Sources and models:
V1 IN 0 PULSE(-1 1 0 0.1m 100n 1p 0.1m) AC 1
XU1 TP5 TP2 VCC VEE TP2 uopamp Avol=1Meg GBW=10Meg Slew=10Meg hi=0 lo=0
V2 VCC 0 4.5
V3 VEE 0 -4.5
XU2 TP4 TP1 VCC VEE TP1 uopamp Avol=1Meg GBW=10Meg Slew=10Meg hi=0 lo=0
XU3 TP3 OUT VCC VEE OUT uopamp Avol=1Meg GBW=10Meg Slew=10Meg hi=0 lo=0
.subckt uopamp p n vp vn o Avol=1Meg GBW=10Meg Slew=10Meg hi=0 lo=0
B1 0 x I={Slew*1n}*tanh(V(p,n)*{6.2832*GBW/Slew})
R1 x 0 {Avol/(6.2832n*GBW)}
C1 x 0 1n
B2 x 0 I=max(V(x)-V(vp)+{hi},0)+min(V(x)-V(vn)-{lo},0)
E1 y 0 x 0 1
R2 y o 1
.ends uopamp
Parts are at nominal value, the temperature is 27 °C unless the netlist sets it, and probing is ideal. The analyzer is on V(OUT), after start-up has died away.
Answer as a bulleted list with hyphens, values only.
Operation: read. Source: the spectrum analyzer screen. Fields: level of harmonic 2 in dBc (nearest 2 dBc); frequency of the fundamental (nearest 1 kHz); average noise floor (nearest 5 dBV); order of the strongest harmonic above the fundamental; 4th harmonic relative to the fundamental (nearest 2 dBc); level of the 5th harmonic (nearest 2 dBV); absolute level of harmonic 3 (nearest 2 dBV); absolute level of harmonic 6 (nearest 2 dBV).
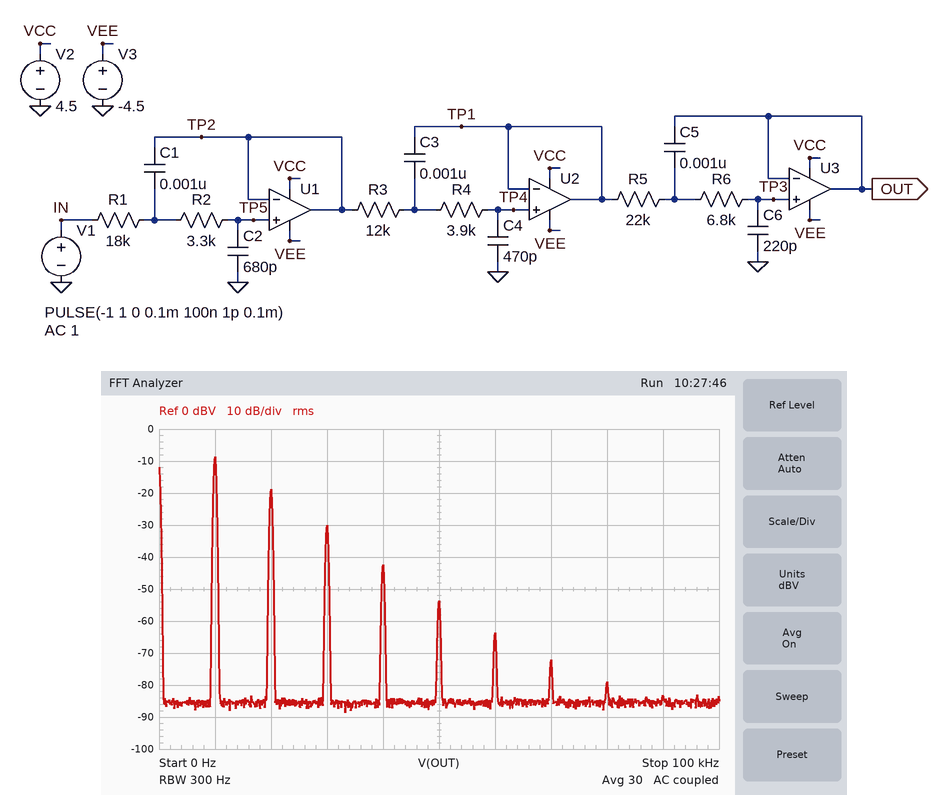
- -10 dBc
- 10 kHz
- -85 dBV
- 2
- -34 dBc
- -54 dBV
- -30 dBV
- -64 dBV
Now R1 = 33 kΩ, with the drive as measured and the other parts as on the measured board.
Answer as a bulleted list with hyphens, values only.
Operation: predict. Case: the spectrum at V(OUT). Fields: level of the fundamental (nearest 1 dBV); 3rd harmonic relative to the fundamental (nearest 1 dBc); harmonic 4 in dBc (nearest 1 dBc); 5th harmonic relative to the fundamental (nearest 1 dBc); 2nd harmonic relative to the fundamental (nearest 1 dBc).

- -11 dBV
- -24 dBc
- -36 dBc
- -48 dBc
- -12 dBc
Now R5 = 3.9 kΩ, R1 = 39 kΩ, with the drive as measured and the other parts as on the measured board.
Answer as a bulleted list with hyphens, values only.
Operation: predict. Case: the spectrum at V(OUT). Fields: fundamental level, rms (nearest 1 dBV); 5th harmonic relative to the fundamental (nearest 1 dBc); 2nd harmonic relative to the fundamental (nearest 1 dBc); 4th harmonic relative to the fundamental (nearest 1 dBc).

- -13 dBV
- -37 dBc
- -12 dBc
- -29 dBc
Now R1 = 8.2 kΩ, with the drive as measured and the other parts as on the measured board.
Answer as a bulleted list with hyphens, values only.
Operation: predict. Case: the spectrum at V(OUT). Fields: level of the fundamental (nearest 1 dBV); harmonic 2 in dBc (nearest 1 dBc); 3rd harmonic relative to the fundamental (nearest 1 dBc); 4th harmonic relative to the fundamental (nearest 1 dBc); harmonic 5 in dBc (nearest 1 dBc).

- -7 dBV
- -8 dBc
- -18 dBc
- -29 dBc
- -40 dBc
